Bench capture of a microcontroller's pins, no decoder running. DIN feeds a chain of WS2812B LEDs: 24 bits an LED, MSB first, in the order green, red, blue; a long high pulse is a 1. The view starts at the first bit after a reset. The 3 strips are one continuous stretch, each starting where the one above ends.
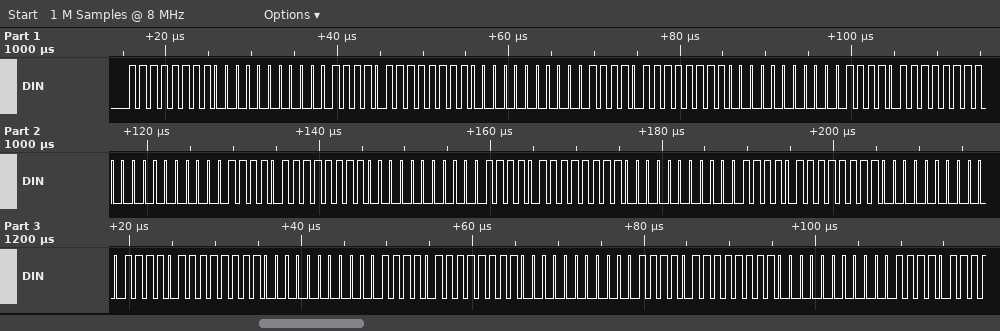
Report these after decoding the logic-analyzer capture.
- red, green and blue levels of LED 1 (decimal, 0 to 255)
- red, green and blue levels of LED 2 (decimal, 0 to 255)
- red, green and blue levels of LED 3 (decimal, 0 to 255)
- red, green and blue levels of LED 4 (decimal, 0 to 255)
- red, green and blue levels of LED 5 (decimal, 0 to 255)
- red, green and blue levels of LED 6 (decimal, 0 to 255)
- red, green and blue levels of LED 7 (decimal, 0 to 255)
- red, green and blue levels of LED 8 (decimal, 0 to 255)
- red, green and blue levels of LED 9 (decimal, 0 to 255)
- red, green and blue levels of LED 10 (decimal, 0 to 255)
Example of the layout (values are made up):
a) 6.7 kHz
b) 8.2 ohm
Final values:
a) 0, 255, 30
b) 0, 255, 30
c) 0, 255, 30
d) 0, 255, 30
e) 0, 255, 30
f) 0, 255, 30
g) 0, 255, 30
h) 0, 255, 30
i) 0, 255, 30
j) 0, 255, 30
